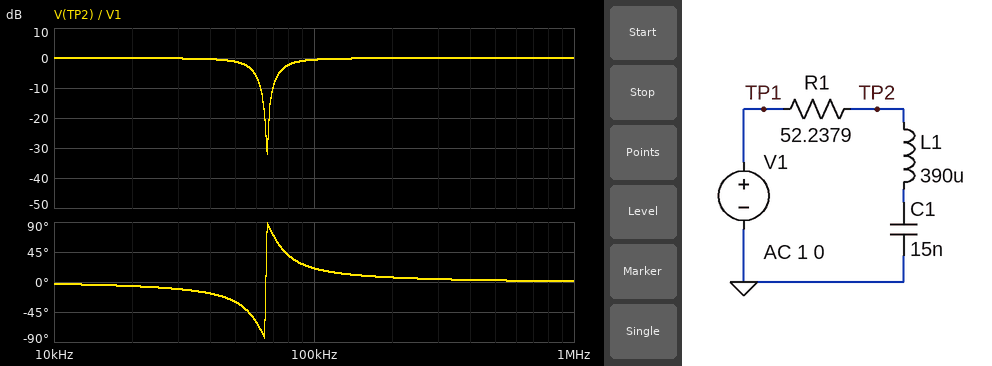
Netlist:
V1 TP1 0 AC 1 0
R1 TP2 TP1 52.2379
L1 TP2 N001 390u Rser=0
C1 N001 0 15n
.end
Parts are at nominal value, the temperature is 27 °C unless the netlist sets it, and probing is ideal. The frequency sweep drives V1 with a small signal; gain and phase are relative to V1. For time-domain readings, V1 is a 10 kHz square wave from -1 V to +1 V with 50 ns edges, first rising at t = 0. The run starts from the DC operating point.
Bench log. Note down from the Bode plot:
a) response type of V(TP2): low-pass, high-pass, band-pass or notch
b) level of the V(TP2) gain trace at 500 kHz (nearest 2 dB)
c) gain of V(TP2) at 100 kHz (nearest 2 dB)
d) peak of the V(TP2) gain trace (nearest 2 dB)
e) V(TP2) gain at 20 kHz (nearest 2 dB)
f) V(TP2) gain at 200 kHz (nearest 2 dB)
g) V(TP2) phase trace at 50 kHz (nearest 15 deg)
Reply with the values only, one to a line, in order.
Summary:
notch
0 dB
0 dB
0 dB
0 dB
0 dB
-30 deg
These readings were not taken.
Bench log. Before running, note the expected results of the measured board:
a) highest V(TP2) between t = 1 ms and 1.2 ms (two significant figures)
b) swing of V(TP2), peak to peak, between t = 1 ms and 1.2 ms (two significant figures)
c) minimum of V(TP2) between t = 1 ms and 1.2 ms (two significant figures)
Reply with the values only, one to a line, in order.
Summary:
1.3 V
2.6 V
-1.3 V
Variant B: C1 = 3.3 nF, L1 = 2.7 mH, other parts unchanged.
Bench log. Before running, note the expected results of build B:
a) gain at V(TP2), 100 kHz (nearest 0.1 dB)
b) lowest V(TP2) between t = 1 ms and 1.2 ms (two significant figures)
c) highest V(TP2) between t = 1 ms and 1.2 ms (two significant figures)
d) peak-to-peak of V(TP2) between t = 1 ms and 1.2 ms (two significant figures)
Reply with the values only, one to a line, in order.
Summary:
0 dB
-1.1 V
1.1 V
2.2 V
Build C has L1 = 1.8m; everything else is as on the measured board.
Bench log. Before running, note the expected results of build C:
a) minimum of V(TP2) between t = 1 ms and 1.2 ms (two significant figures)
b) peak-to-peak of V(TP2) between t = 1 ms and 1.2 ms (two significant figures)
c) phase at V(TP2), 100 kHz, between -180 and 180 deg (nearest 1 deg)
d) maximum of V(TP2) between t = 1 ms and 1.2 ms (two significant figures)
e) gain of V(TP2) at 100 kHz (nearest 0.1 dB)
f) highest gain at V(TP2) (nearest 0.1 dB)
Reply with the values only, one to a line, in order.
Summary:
-1.4 V
2.8 V
3 deg
1.4 V
0 dB
0 dB
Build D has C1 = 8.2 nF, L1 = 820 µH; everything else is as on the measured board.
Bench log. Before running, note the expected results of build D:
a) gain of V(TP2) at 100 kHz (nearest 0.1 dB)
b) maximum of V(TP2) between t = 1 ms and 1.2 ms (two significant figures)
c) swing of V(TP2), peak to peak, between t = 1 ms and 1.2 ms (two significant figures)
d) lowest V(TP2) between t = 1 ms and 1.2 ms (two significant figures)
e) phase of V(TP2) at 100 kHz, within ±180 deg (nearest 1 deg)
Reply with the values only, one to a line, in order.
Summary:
-0.1 dB
1.2 V
2.4 V
-1.2 V
9 deg
